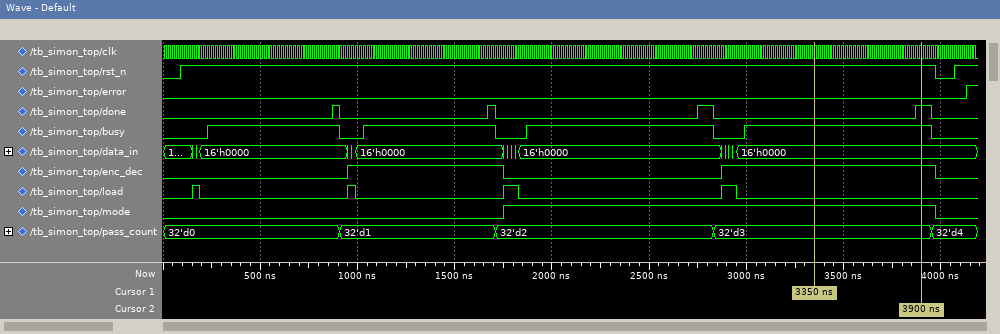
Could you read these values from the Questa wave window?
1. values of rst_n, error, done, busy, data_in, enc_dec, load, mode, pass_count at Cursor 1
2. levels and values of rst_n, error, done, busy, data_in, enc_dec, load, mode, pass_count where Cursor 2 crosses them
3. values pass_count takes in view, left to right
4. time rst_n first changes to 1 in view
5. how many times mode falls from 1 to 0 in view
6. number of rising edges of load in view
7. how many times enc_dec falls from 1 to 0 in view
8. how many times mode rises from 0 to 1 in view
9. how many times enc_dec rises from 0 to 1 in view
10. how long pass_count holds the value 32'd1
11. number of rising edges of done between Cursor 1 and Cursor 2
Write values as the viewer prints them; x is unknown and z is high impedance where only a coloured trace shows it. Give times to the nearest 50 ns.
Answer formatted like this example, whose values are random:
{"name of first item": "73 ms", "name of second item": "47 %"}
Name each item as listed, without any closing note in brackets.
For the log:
{"values of rst_n, error, done, busy, data_in, enc_dec, load, mode, pass_count at Cursor 1": "rst_n=1, error=0, done=0, busy=1, data_in=16'h0000, enc_dec=1, load=0, mode=1, pass_count=32'd3", "levels and values of rst_n, error, done, busy, data_in, enc_dec, load, mode, pass_count where Cursor 2 crosses them": "rst_n=1, error=0, done=1, busy=1, data_in=16'h0000, enc_dec=1, load=0, mode=1, pass_count=32'd3", "values pass_count takes in view, left to right": "32'd0, 32'd1, 32'd2, 32'd3, 32'd4", "time rst_n first changes to 1 in view": "100 ns", "how many times mode falls from 1 to 0 in view": "1", "number of rising edges of load in view": "4", "how many times enc_dec falls from 1 to 0 in view": "2", "how many times mode rises from 0 to 1 in view": "1", "how many times enc_dec rises from 0 to 1 in view": "2", "how long pass_count holds the value 32'd1": "800 ns", "number of rising edges of done between Cursor 1 and Cursor 2": "1"}
